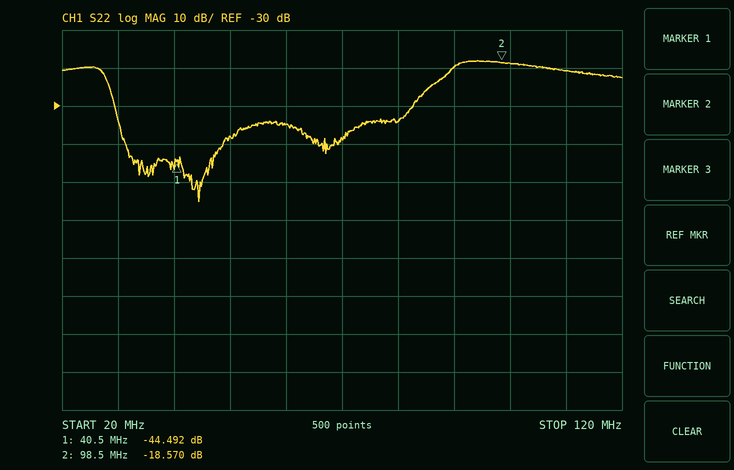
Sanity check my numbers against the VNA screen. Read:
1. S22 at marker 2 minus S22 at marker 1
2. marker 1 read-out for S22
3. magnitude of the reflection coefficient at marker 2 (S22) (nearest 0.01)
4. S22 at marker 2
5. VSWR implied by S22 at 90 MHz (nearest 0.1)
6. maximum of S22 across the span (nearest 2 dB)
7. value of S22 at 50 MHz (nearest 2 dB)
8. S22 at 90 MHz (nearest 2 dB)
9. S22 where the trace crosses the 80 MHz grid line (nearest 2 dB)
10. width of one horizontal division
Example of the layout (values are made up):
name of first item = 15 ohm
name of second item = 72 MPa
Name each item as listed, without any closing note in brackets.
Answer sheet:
S22 at marker 2 minus S22 at marker 1 = 25.922 dB
marker 1 read-out for S22 = -44.492 dB
magnitude of the reflection coefficient at marker 2 (S22) = 0.12
S22 at marker 2 = -18.570 dB
VSWR implied by S22 at 90 MHz = 1.2
maximum of S22 across the span = -18 dB
value of S22 at 50 MHz = -38 dB
S22 at 90 MHz = -20 dB
S22 where the trace crosses the 80 MHz grid line = -34 dB
width of one horizontal division = 10 MHz
